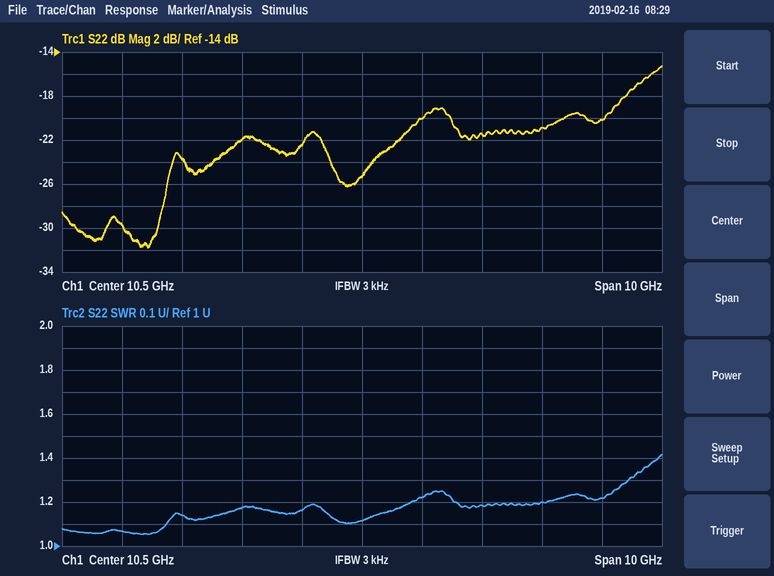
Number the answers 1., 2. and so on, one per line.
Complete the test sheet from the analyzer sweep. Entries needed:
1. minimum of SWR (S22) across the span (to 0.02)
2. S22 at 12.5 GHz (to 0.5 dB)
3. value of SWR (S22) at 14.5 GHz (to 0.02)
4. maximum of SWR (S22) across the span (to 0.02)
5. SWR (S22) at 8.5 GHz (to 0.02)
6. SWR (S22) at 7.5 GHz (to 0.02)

1. 1.06
2. -21.5 dB
3. 1.22
4. 1.42
5. 1.18
6. 1.14
